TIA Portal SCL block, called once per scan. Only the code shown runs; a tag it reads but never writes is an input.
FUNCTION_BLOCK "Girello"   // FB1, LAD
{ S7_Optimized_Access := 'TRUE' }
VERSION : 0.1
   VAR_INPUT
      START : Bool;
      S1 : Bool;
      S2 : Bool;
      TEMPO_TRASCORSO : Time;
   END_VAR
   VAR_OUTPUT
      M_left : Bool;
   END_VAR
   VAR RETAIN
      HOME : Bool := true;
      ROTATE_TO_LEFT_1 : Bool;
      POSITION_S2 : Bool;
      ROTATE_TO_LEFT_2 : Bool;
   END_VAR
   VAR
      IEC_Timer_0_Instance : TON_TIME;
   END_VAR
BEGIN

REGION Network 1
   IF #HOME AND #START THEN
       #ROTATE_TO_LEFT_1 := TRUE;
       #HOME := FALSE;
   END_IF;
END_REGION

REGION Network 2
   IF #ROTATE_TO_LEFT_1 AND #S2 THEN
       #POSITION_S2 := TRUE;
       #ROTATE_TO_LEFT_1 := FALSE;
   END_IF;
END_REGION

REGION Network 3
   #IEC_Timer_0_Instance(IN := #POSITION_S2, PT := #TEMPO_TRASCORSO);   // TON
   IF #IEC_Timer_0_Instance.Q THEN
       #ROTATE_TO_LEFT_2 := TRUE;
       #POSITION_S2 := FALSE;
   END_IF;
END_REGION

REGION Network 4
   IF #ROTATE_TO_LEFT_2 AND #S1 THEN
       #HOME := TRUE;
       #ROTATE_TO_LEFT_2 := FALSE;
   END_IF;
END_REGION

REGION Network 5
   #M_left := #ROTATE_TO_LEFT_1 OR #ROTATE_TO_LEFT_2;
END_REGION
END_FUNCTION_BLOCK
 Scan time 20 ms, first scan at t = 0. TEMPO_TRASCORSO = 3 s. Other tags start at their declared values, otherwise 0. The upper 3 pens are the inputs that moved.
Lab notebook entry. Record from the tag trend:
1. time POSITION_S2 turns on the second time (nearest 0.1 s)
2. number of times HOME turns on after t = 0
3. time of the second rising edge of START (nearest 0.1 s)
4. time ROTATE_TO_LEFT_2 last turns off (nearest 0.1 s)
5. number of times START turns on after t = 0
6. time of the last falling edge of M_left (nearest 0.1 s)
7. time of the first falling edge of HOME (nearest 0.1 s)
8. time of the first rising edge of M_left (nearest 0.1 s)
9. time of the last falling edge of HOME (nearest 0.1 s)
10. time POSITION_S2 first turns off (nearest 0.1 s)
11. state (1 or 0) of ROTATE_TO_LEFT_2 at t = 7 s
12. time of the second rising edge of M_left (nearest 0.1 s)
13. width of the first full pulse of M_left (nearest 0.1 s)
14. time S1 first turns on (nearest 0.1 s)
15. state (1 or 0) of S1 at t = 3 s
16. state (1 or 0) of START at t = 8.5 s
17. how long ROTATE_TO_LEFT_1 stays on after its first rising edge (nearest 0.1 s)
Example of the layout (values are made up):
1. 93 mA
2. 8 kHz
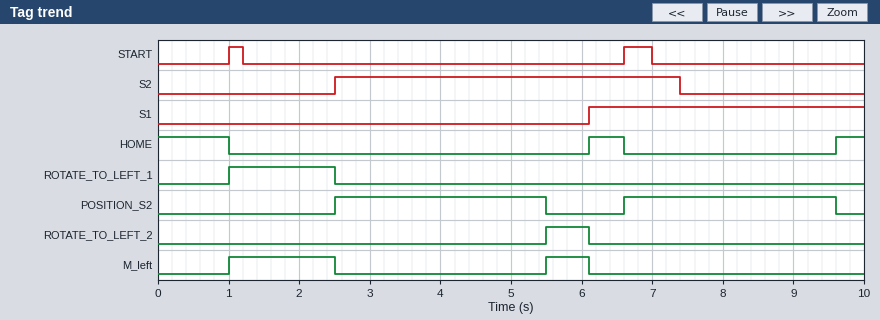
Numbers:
1. 6.6 s
2. 2
3. 6.6 s
4. 6.1 s
5. 2
6. 6.1 s
7. 1.0 s
8. 1.0 s
9. 6.6 s
10. 5.5 s
11. 0
12. 5.5 s
13. 1.5 s
14. 6.1 s
15. 0
16. 0
17. 1.5 s
